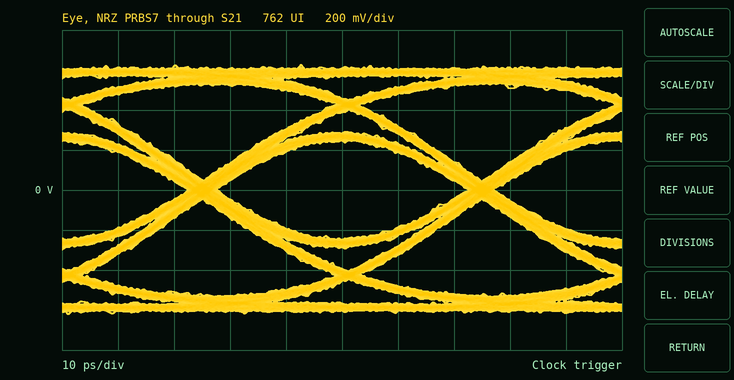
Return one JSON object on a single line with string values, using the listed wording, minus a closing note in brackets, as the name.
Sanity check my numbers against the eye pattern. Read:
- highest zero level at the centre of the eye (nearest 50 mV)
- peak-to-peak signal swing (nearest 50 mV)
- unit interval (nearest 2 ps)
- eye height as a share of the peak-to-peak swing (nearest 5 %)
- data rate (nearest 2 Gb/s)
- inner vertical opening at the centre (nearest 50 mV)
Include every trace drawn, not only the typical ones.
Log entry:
{"highest zero level at the centre of the eye": "-250 mV", "peak-to-peak signal swing": "1.25 V", "unit interval": "50 ps", "eye height as a share of the peak-to-peak swing": "40 %", "data rate": "20 Gb/s", "inner vertical opening at the centre": "500 mV"}
